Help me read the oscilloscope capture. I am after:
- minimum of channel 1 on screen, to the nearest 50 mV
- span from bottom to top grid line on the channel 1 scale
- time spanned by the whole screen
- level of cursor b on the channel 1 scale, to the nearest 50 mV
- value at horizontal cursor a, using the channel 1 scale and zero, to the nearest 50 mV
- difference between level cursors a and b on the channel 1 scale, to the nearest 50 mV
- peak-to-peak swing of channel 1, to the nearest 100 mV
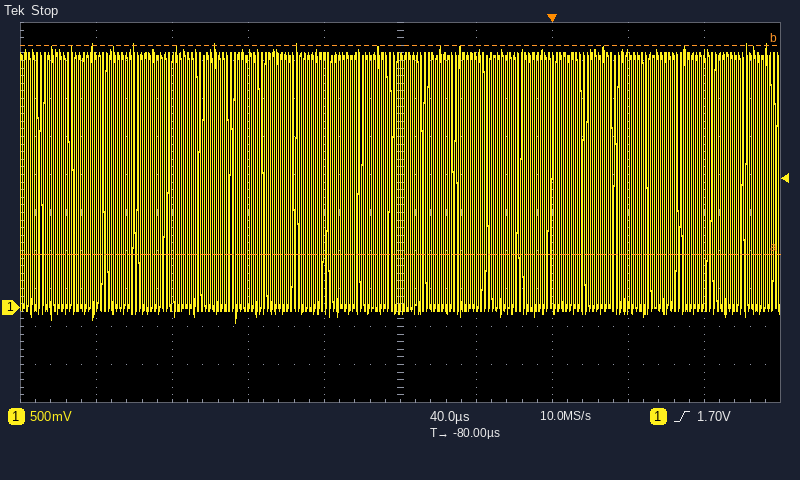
-200 mV
5 V
400 µs
3.45 V
700 mV
2.75 V
3.70 V
